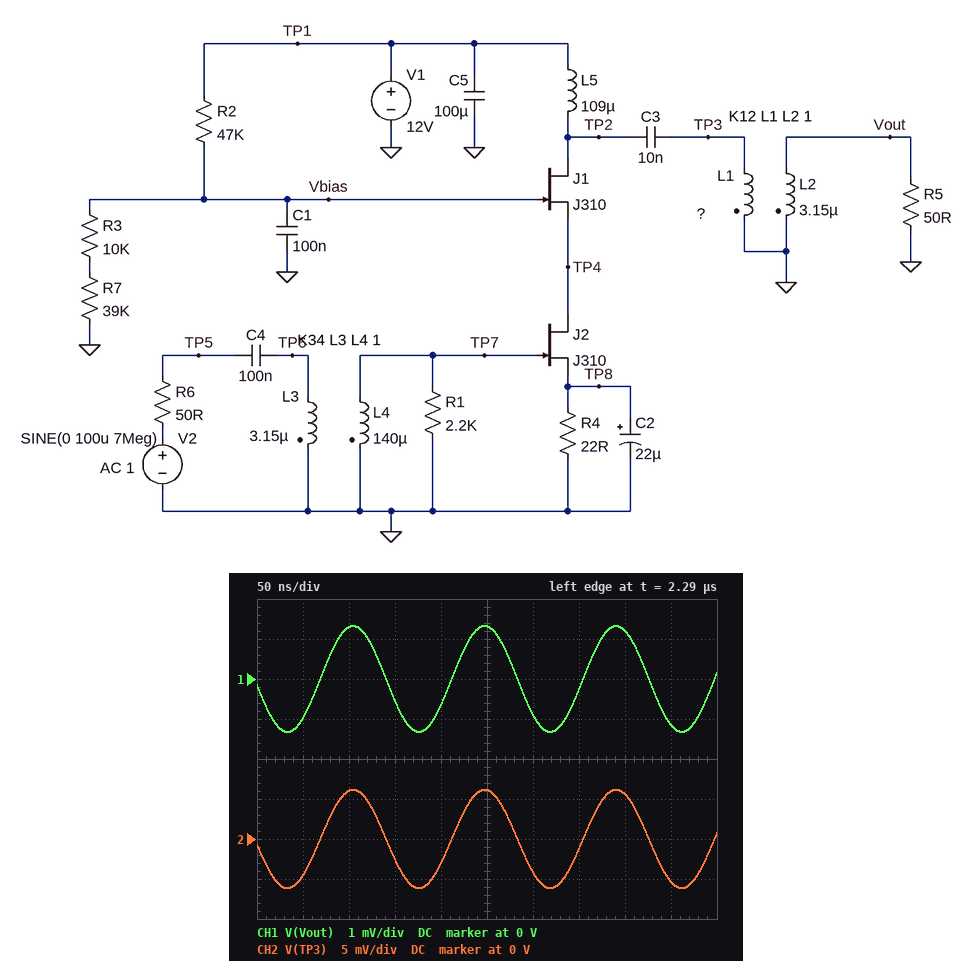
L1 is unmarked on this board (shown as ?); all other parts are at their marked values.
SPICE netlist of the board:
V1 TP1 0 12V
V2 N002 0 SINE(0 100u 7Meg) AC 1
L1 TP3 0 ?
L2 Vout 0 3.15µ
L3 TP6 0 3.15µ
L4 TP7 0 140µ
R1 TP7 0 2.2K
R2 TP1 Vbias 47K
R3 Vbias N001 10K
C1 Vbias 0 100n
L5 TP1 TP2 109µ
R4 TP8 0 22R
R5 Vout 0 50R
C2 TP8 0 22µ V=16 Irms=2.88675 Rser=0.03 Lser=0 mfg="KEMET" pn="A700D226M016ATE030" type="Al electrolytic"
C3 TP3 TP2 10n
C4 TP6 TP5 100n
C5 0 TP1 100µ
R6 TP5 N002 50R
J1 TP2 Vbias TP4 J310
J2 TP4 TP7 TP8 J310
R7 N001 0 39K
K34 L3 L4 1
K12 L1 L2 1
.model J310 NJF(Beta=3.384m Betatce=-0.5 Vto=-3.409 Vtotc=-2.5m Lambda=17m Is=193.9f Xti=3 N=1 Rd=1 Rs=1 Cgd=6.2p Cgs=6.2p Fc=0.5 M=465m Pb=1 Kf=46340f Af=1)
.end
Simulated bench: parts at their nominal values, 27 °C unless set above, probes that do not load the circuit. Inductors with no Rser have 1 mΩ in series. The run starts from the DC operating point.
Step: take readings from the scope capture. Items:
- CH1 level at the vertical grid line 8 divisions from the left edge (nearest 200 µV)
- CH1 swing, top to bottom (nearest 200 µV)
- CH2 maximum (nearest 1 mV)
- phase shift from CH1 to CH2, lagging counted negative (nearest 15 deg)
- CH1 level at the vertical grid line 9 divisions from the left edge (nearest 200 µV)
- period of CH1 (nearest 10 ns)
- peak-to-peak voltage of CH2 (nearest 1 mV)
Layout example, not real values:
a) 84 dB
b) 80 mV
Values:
a) 1.2 mV
b) 2.6 mV
c) 6 mV
d) 0 deg
e) -1.2 mV
f) 140 ns
g) 12 mV
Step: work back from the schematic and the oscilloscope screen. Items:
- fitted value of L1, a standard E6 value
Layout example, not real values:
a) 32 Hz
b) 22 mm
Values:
a) 68 µH
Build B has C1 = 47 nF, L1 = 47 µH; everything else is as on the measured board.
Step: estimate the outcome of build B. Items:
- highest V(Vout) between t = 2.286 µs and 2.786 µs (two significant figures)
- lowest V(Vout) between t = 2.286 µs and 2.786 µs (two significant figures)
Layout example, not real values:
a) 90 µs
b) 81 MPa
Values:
a) 1.1 mV
b) -1.1 mV
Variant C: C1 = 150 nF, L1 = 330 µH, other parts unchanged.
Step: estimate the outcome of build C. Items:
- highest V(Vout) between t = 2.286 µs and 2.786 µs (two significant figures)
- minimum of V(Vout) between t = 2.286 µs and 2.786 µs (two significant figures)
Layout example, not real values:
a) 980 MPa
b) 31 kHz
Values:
a) 2.5 mV
b) -2.5 mV
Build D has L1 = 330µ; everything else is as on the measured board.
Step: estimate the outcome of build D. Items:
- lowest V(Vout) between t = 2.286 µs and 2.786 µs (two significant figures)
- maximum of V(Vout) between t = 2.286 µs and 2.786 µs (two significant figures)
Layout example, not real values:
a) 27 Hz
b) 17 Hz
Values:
a) -2.5 mV
b) 2.5 mV
